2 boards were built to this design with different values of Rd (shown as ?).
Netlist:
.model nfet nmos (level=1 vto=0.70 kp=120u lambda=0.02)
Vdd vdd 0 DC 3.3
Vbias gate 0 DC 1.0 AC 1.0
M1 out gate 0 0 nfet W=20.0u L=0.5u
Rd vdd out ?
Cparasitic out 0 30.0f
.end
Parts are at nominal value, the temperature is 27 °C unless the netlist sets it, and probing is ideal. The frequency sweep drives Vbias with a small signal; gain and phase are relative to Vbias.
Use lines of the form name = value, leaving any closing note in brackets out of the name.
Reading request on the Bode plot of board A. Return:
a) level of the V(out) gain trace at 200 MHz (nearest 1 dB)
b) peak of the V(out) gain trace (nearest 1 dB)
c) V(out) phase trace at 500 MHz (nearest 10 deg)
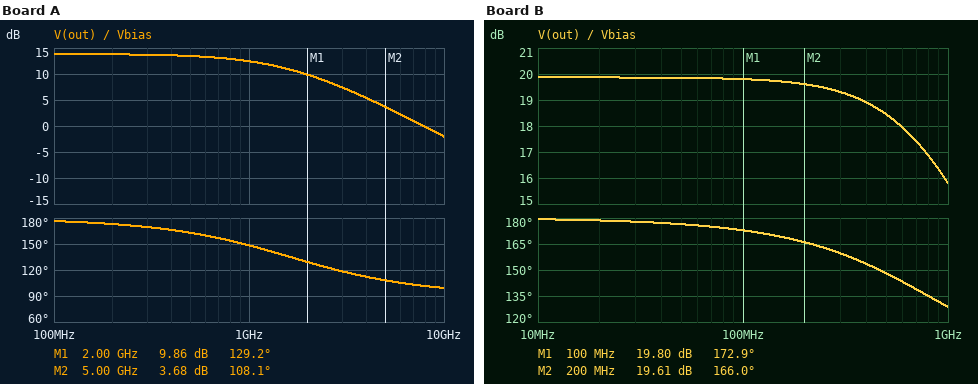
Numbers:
level of the V(out) gain trace at 200 MHz = 14 dB
peak of the V(out) gain trace = 14 dB
V(out) phase trace at 500 MHz = 160 deg
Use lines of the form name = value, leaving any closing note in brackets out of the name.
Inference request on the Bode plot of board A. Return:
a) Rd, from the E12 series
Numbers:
Rd, from the E12 series = 3.3 kΩ
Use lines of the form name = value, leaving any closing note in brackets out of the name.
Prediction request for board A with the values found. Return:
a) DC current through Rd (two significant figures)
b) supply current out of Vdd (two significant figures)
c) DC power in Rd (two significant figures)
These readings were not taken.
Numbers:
DC current through Rd = 230 µA
supply current out of Vdd = 230 µA
DC power in Rd = 170 µW
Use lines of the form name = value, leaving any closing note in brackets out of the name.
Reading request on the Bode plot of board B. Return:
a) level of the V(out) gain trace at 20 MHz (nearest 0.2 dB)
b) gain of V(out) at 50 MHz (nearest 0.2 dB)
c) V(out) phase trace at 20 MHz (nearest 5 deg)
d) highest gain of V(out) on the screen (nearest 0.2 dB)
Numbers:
level of the V(out) gain trace at 20 MHz = 19.8 dB
gain of V(out) at 50 MHz = 19.8 dB
V(out) phase trace at 20 MHz = 180 deg
highest gain of V(out) on the screen = 19.8 dB
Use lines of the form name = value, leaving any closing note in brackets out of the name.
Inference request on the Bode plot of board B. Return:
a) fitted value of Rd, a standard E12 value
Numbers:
fitted value of Rd, a standard E12 value = 6.8 kΩ
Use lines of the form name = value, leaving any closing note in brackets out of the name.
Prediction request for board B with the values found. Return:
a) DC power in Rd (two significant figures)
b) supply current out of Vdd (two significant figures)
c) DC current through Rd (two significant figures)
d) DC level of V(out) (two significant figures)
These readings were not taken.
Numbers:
DC power in Rd = 340 µW
supply current out of Vdd = 220 µA
DC current through Rd = 220 µA
DC level of V(out) = 1.8 V
